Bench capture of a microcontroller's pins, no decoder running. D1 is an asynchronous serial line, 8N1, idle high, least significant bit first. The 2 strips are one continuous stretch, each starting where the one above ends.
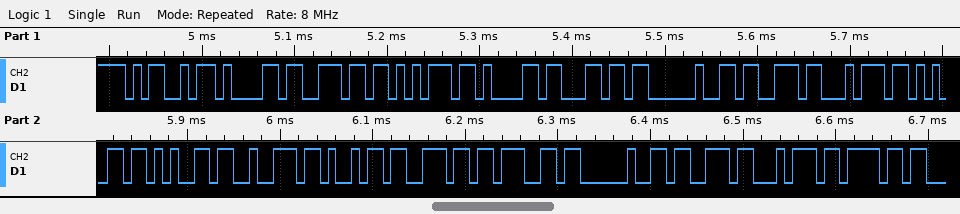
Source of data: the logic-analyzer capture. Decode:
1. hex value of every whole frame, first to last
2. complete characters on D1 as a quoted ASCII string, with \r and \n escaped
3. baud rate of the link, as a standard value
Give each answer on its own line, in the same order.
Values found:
4D 61 6E 75 61 6C 20 73 74 65 65 72 69 6E 67 20 73 74 6F
"Manual steering sto"
115200 baud
